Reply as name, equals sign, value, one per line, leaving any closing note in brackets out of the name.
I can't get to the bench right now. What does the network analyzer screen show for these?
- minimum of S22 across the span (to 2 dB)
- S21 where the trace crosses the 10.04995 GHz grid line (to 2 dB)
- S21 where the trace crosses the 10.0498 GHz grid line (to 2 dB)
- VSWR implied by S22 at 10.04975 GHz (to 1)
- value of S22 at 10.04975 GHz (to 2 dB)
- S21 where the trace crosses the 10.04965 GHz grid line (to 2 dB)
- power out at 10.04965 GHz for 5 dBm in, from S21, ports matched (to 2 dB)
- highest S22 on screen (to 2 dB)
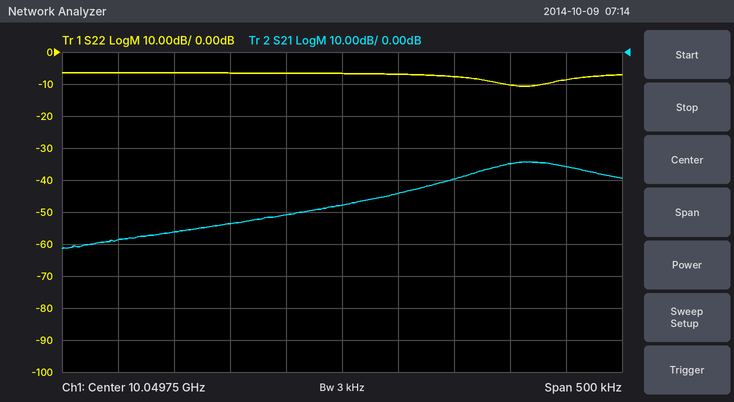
minimum of S22 across the span = -10 dB
S21 where the trace crosses the 10.04995 GHz grid line = -36 dB
S21 where the trace crosses the 10.0498 GHz grid line = -44 dB
VSWR implied by S22 at 10.04975 GHz = 3
value of S22 at 10.04975 GHz = -6 dB
S21 where the trace crosses the 10.04965 GHz grid line = -54 dB
power out at 10.04965 GHz for 5 dBm in, from S21, ports matched = -48 dBm
highest S22 on screen = -6 dB
